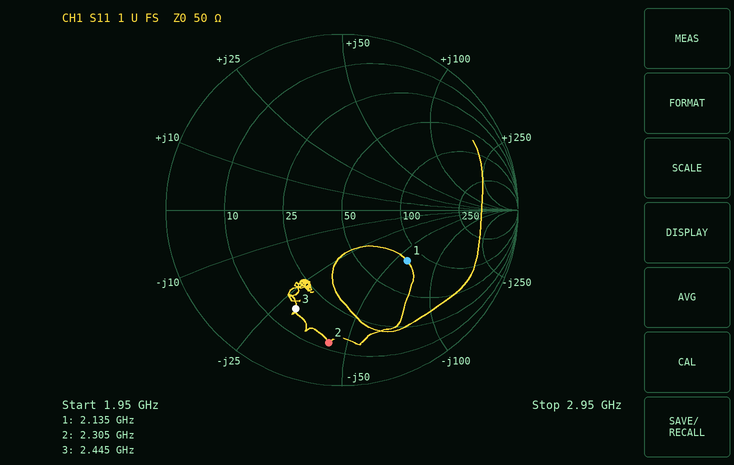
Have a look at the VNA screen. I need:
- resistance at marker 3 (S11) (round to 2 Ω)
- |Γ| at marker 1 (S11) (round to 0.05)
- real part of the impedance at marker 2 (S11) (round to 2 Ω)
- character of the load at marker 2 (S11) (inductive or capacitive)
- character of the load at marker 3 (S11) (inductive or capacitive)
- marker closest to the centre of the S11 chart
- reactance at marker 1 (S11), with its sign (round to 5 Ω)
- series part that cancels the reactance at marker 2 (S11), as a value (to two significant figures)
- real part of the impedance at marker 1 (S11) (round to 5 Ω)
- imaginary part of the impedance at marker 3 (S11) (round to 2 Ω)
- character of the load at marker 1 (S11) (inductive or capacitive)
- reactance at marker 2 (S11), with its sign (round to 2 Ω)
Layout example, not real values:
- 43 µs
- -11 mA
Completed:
- 16 Ω
- 0.45
- 12 Ω
- capacitive
- capacitive
- marker 1
- -60 Ω
- 3.0 nH
- 80 Ω
- -30 Ω
- capacitive
- -44 Ω
